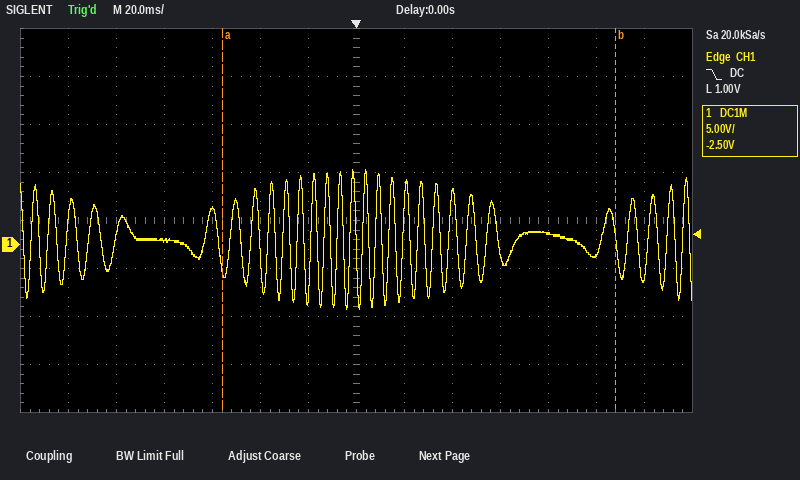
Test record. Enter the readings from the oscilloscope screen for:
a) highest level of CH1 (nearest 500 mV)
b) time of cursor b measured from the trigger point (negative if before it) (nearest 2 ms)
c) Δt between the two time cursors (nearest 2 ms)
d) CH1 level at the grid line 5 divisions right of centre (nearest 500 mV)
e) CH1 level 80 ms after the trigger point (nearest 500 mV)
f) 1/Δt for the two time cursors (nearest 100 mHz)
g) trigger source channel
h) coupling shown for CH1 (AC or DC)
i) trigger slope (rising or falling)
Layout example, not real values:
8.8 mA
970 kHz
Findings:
8.0 V
+108 ms
164 ms
-1.0 V
1.0 V
6.1 Hz
CH1
DC
falling
